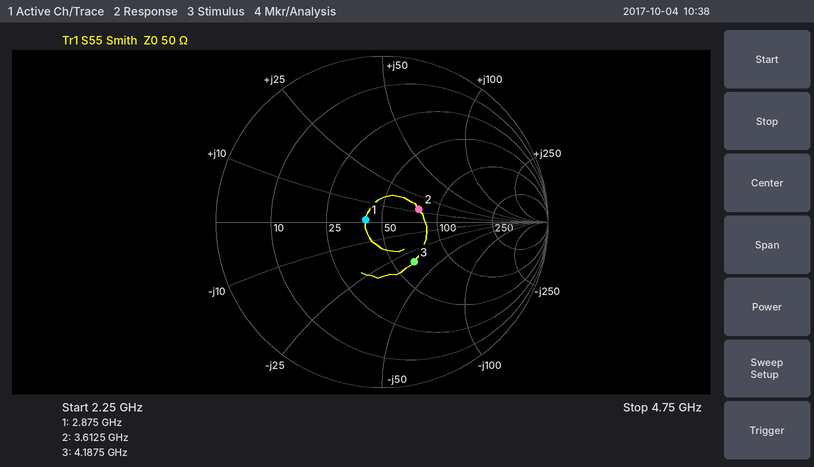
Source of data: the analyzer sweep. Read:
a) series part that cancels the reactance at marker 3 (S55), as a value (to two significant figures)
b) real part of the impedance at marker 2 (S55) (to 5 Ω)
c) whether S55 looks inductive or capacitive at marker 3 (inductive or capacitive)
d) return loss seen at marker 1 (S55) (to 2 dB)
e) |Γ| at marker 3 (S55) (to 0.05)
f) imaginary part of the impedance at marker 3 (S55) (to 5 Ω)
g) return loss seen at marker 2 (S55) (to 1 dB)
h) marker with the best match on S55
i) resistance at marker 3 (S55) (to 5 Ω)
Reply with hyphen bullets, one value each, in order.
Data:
- 1.3 nH
- 75 Ω
- capacitive
- 20 dB
- 0.30
- -35 Ω
- 13 dB
- marker 1
- 65 Ω
